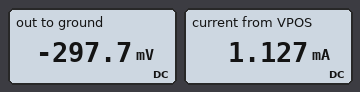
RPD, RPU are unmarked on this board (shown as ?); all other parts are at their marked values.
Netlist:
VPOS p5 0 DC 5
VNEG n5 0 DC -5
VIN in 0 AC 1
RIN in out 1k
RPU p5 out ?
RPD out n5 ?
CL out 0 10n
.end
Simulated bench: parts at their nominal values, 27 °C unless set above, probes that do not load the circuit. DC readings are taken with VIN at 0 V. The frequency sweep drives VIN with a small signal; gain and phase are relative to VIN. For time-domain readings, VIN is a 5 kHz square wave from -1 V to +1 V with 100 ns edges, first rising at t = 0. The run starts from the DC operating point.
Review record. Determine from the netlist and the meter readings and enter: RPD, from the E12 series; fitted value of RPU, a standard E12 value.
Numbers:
3.3 kΩ
4.7 kΩ
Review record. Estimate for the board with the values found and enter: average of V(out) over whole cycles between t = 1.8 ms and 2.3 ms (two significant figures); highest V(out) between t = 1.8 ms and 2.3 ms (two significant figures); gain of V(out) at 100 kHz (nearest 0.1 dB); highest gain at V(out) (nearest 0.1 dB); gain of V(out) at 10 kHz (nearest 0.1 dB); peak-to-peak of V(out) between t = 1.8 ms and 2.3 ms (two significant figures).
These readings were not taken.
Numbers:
-300 mV
360 mV
-16.2 dB
-3.6 dB
-4.3 dB
1.3 V
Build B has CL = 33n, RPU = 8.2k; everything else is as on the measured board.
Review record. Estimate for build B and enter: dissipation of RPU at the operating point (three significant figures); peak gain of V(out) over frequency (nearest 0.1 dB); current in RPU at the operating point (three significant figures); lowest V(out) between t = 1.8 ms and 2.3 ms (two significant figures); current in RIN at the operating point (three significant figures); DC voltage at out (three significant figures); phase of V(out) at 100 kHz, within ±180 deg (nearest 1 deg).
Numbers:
3.87 mW
-3.1 dB
687 µA
-1.3 V
635 µA
-635 mV
-86 deg
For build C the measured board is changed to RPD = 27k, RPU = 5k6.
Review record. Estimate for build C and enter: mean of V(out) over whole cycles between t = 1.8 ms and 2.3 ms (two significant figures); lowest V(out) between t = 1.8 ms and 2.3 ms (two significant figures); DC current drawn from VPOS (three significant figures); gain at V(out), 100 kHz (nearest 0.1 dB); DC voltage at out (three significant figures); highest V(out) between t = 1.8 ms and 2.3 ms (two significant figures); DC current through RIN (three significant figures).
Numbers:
580 mV
-240 mV
789 µA
-16.1 dB
582 mV
1.4 V
582 µA
